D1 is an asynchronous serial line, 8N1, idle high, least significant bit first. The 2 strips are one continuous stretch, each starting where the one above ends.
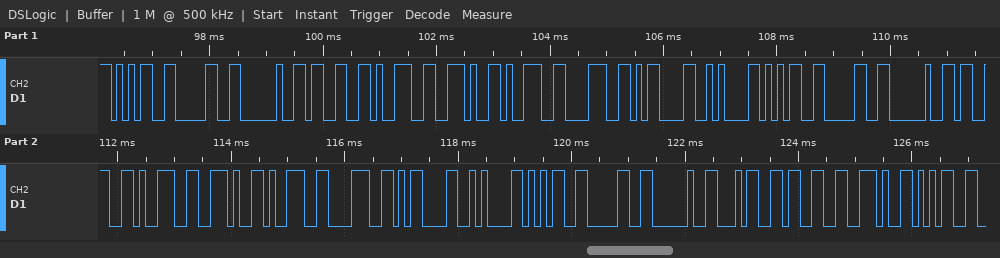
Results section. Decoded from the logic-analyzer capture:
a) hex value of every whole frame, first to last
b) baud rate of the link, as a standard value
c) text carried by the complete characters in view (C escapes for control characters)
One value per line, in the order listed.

35 30 20 33 39 2E 39 38 0D 0A 35 30 20 33 39 2E 39 38 0D 0A 35 30 20 34 33 2E 35
9600 baud
"50 39.98\r\n50 39.98\r\n50 43.5"
